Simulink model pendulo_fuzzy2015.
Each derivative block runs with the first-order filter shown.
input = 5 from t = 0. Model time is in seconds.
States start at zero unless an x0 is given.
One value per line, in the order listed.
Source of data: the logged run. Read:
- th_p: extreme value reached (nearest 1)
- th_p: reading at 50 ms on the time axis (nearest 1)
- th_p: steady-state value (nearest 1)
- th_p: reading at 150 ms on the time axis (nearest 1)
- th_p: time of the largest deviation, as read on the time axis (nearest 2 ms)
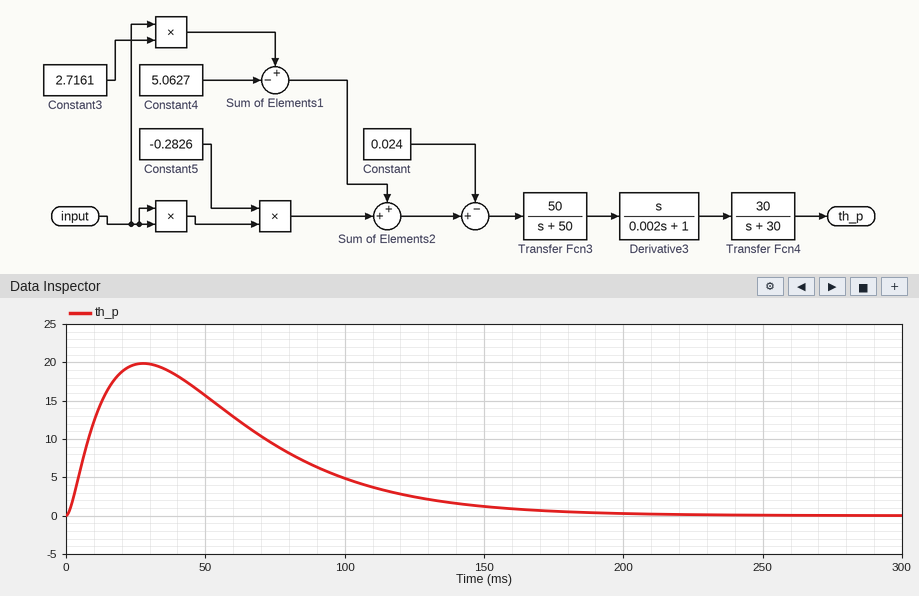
20
16
0
1
28 ms
